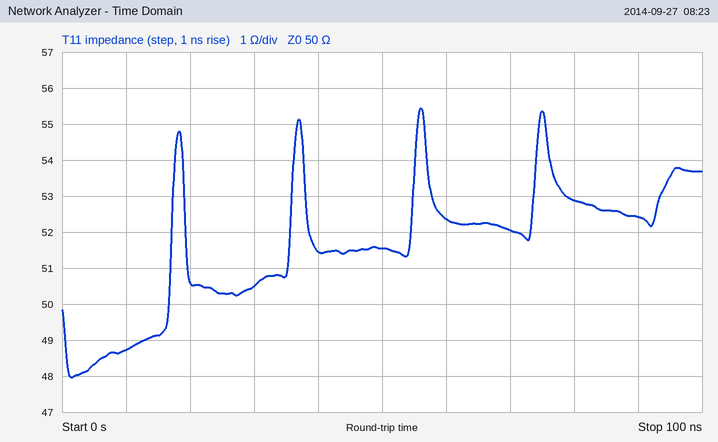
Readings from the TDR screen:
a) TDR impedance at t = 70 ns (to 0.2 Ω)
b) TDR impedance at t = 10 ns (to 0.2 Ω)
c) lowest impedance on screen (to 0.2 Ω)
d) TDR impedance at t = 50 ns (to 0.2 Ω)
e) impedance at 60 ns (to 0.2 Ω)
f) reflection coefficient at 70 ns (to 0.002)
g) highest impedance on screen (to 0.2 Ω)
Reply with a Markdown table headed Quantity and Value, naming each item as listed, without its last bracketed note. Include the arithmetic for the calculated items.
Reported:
| Quantity | Value |
|---|---|
| TDR impedance at t = 70 ns | 52.0 Ω |
| TDR impedance at t = 10 ns | 48.8 Ω |
| lowest impedance on screen | 48.0 Ω |
| TDR impedance at t = 50 ns | 51.6 Ω |
| impedance at 60 ns | 52.4 Ω |
| reflection coefficient at 70 ns | (52 − 50)/(52 + 50) ≈ +0.020 |
| highest impedance on screen | 55.4 Ω |
